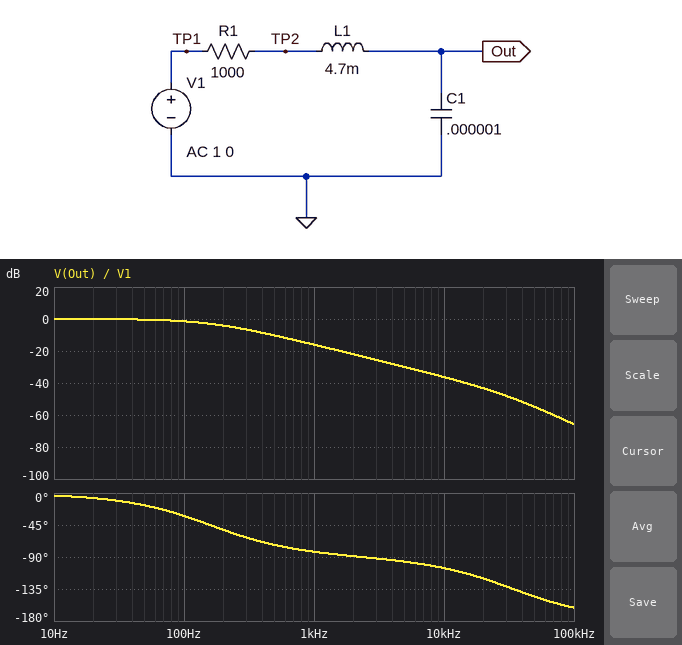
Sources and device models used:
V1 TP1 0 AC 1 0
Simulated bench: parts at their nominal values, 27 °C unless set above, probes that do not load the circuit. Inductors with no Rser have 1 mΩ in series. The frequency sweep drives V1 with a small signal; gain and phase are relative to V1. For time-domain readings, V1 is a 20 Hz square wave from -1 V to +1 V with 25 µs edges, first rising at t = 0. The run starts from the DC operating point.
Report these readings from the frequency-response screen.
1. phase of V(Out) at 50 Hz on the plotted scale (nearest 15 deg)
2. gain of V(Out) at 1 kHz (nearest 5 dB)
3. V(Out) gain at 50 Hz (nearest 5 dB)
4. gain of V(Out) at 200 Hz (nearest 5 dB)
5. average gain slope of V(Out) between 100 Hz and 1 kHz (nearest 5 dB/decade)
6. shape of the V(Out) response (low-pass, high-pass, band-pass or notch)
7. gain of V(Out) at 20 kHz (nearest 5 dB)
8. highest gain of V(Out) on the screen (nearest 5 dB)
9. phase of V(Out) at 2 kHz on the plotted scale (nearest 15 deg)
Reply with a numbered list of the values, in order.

1. -15 deg
2. -15 dB
3. 0 dB
4. -5 dB
5. -15 dB/decade
6. low-pass
7. -45 dB
8. 0 dB
9. -90 deg
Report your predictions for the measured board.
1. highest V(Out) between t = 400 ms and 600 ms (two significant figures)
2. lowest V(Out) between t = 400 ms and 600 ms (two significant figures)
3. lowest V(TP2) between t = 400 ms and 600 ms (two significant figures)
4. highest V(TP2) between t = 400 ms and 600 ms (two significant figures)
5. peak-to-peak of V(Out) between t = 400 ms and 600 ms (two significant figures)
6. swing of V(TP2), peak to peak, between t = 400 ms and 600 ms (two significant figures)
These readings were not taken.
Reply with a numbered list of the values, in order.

1. 1.0 V
2. -1.0 V
3. -1.0 V
4. 1.0 V
5. 2.0 V
6. 2.0 V
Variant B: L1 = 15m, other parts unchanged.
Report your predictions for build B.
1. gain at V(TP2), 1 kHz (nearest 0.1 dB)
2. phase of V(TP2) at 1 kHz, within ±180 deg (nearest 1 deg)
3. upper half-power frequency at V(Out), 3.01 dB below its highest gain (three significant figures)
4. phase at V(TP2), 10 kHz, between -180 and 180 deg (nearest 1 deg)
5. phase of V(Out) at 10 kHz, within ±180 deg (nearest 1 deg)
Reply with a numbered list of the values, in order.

1. -23.8 dB
2. -86 deg
3. 162 Hz
4. 47 deg
5. -133 deg
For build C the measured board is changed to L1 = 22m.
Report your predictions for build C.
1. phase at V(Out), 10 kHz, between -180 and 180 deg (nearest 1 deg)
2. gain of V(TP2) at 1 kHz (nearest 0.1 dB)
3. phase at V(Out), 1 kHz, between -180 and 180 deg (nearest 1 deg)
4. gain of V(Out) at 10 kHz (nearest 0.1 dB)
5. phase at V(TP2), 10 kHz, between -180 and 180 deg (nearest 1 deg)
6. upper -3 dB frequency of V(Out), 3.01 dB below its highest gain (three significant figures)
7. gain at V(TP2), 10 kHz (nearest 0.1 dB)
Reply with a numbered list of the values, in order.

1. -144 deg
2. -33.6 dB
3. -89 deg
4. -40.5 dB
5. 36 deg
6. 163 Hz
7. -1.9 dB
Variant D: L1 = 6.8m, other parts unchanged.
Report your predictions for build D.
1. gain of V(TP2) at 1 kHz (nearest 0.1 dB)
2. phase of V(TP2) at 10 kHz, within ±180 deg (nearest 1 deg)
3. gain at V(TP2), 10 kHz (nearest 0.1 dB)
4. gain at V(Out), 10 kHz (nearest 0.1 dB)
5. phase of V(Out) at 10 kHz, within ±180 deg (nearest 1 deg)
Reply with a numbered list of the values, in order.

1. -18.7 dB
2. 68 deg
3. -8.4 dB
4. -36.6 dB
5. -112 deg
